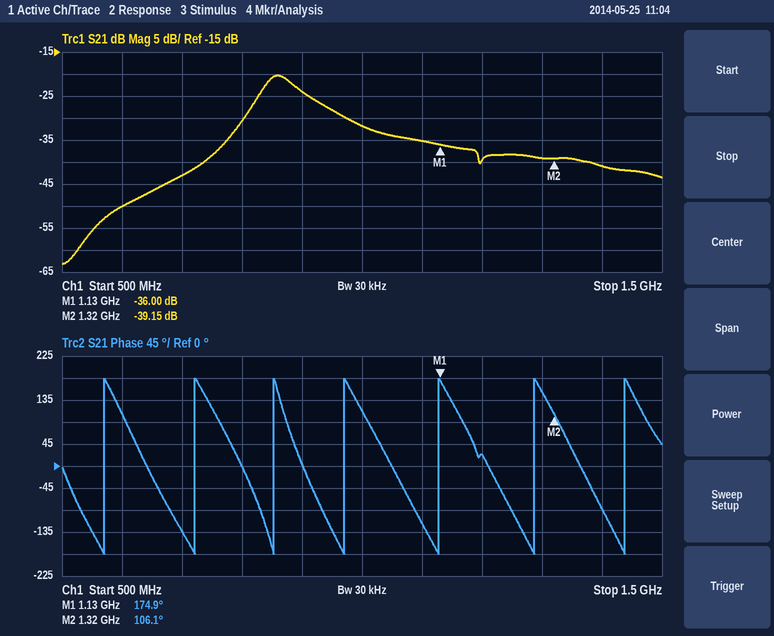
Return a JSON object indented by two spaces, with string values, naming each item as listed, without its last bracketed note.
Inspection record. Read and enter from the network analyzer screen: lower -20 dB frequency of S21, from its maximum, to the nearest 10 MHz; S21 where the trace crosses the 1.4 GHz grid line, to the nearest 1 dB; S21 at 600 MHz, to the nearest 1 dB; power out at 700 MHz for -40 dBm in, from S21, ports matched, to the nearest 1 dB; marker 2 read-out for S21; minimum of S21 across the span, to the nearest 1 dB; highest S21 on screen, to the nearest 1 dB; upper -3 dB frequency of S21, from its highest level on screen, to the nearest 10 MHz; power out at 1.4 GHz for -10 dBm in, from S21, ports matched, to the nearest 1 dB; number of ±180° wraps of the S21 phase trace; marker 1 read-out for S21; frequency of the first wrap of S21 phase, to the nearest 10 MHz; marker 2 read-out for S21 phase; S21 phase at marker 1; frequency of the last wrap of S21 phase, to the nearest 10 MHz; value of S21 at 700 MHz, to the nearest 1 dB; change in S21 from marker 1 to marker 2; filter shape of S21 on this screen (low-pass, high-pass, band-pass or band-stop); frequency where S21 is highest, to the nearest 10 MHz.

{
  "lower -20 dB frequency of S21, from its maximum, to the nearest 10 MHz": "730 MHz",
  "S21 where the trace crosses the 1.4 GHz grid line, to the nearest 1 dB": "-41 dB",
  "S21 at 600 MHz, to the nearest 1 dB": "-50 dB",
  "power out at 700 MHz for -40 dBm in, from S21, ports matched, to the nearest 1 dB": "-83 dBm",
  "marker 2 read-out for S21": "-39.15 dB",
  "minimum of S21 across the span, to the nearest 1 dB": "-63 dB",
  "highest S21 on screen, to the nearest 1 dB": "-20 dB",
  "upper -3 dB frequency of S21, from its highest level on screen, to the nearest 10 MHz": "890 MHz",
  "power out at 1.4 GHz for -10 dBm in, from S21, ports matched, to the nearest 1 dB": "-51 dBm",
  "number of ±180° wraps of the S21 phase trace": "7",
  "marker 1 read-out for S21": "-36.00 dB",
  "frequency of the first wrap of S21 phase, to the nearest 10 MHz": "570 MHz",
  "marker 2 read-out for S21 phase": "106.1°",
  "S21 phase at marker 1": "174.9°",
  "frequency of the last wrap of S21 phase, to the nearest 10 MHz": "1.44 GHz",
  "value of S21 at 700 MHz, to the nearest 1 dB": "-43 dB",
  "change in S21 from marker 1 to marker 2": "-3.15 dB",
  "filter shape of S21 on this screen": "band-pass",
  "frequency where S21 is highest, to the nearest 10 MHz": "860 MHz"
}
